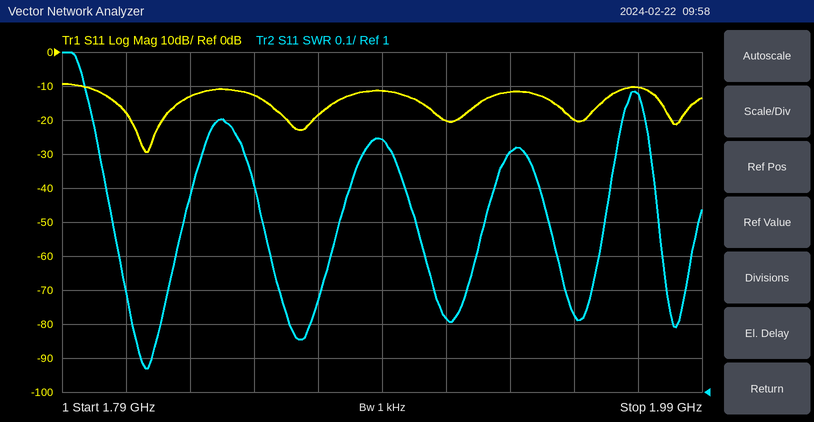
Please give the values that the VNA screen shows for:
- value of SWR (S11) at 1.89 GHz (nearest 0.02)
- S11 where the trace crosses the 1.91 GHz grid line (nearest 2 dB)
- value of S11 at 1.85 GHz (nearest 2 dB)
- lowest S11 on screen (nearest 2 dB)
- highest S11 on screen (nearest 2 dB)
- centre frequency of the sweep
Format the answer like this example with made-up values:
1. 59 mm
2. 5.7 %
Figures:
1. 1.74
2. -20 dB
3. -12 dB
4. -30 dB
5. -10 dB
6. 1.89 GHz
